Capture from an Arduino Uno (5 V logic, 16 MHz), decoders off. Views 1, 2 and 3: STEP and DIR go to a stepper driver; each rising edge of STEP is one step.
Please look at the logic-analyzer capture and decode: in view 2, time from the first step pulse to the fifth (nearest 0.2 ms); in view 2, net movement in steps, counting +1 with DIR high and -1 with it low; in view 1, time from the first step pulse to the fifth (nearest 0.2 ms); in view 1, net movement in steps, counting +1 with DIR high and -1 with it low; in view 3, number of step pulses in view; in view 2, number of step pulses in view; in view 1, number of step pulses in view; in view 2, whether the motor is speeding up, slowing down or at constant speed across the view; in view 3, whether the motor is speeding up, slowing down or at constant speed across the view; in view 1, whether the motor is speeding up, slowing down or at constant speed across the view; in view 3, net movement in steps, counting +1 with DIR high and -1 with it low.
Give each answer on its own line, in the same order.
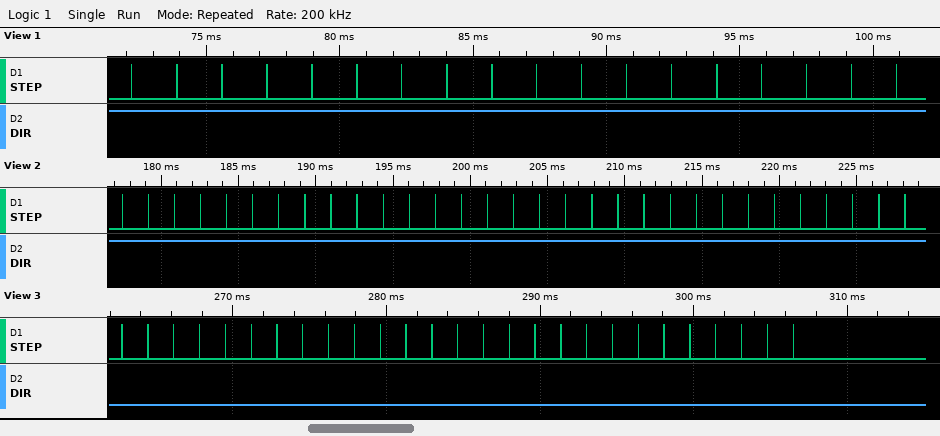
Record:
6.8 ms
+31
6.8 ms
+18
27
31
18
constant speed
constant speed
constant speed
-27
